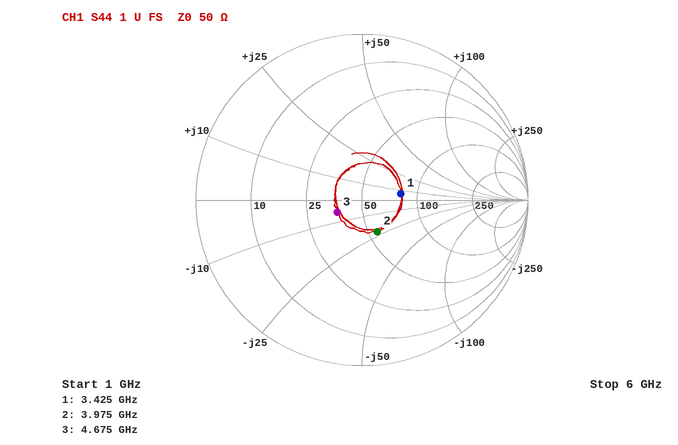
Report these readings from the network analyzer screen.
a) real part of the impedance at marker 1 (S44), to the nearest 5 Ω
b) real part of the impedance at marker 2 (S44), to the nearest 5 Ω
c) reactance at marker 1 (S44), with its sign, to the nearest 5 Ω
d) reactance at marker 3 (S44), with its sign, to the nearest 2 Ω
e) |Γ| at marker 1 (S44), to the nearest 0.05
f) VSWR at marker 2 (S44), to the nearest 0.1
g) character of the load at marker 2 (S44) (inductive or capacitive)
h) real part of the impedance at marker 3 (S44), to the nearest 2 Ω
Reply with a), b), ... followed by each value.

a) 80 Ω
b) 55 Ω
c) +5 Ω
d) -6 Ω
e) 0.25
f) 1.5
g) capacitive
h) 36 Ω
